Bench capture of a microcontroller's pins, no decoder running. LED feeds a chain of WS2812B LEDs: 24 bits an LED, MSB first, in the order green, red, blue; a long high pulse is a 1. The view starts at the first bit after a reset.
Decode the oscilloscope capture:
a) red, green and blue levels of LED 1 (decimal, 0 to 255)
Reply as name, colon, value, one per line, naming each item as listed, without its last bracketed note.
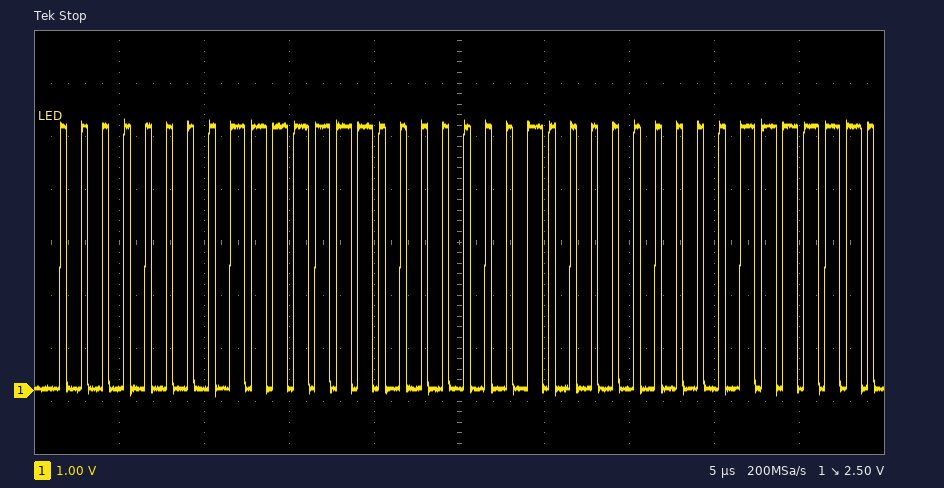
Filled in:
red, green and blue levels of LED 1: 254, 0, 2
